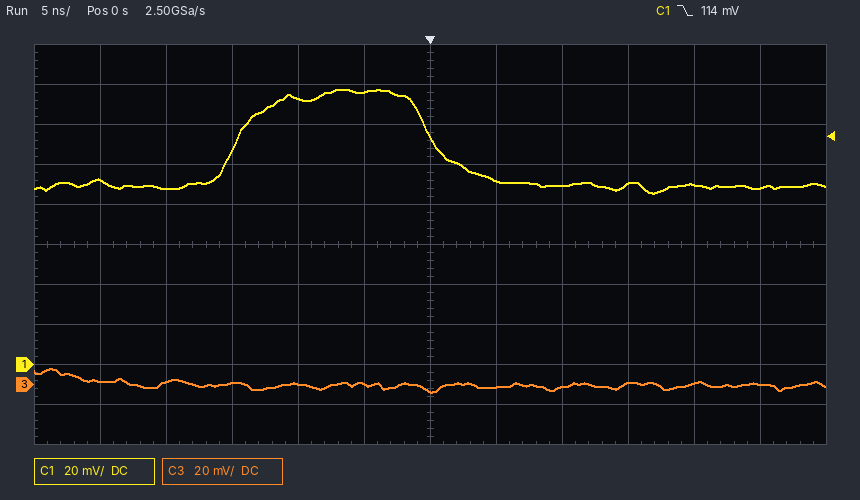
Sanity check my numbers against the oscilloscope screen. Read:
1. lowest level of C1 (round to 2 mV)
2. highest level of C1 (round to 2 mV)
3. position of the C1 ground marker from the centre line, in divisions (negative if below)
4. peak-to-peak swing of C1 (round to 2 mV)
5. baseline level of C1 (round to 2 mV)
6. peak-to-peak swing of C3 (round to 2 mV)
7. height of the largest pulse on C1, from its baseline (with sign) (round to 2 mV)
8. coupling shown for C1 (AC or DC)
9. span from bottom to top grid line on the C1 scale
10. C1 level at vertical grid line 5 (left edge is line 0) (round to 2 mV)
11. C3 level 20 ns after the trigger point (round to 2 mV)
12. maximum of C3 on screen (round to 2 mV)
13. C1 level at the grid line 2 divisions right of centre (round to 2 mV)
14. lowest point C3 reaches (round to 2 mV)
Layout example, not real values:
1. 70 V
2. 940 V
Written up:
1. 86 mV
2. 138 mV
3. -3.0 div
4. 52 mV
5. 90 mV
6. 12 mV
7. +48 mV
8. DC
9. 200 mV
10. 136 mV
11. 0 mV
12. 8 mV
13. 90 mV
14. -4 mV
